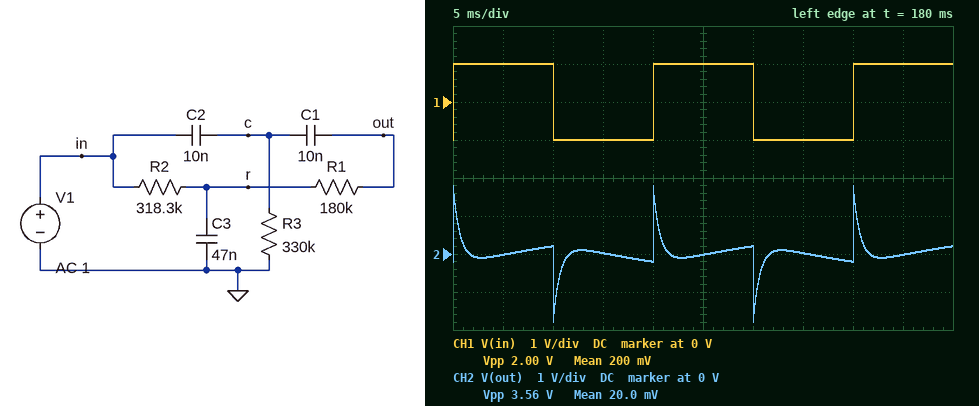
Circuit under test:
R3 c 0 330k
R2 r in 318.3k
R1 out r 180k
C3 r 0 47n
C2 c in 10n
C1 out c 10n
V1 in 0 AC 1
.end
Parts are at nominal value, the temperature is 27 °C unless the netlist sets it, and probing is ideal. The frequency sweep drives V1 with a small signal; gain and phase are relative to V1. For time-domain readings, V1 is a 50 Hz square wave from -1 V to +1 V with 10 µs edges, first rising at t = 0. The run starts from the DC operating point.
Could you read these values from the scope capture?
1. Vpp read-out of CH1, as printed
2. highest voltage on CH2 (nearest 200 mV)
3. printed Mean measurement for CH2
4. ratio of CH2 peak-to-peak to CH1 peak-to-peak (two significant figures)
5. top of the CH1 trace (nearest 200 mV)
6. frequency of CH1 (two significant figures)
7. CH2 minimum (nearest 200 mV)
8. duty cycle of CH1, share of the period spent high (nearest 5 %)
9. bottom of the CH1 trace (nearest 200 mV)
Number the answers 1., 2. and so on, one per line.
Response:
1. 2.00 V
2. 1.8 V
3. 20.0 mV
4. 1.8
5. 1.0 V
6. 50 Hz
7. -1.8 V
8. 50 %
9. -1.0 V
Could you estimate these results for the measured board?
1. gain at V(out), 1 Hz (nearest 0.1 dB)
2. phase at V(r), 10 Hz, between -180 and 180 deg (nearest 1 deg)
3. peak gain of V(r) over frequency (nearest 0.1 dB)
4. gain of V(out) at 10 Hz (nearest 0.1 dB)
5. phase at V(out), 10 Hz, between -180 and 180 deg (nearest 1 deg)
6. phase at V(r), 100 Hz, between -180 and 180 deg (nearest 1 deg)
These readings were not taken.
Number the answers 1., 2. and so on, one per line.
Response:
1. -0.1 dB
2. -46 deg
3. 0 dB
4. -4.5 dB
5. -52 deg
6. -49 deg
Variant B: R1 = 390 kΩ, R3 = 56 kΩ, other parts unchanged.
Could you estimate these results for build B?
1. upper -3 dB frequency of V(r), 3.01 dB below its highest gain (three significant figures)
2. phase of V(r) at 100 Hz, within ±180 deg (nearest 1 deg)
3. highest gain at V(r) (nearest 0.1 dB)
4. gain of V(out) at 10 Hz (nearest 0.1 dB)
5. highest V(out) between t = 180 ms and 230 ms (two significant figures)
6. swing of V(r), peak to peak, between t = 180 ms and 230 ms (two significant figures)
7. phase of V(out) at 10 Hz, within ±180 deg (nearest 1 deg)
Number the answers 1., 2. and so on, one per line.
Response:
1. 8.42 Hz
2. -68 deg
3. 0 dB
4. -4.2 dB
5. 1.9 V
6. 590 mV
7. -61 deg
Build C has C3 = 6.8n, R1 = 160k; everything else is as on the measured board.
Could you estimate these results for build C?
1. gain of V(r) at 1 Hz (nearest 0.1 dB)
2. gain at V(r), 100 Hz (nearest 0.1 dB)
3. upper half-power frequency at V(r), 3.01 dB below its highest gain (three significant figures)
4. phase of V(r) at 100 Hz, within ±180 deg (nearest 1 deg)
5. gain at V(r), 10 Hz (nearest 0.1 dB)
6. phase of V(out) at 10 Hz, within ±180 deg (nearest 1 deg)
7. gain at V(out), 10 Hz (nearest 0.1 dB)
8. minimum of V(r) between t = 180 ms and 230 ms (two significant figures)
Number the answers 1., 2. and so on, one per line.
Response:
1. 0 dB
2. -5.3 dB
3. 22.2 Hz
4. -20 deg
5. -1.1 dB
6. -21 deg
7. -1.5 dB
8. -720 mV
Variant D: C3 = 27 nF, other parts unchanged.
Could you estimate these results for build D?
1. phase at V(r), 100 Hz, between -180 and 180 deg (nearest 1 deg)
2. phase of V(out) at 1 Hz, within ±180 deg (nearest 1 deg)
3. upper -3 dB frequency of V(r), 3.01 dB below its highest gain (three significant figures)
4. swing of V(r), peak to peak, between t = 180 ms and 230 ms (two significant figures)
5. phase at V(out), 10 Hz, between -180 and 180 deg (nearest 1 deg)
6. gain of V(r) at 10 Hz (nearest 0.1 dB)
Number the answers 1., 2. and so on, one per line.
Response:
1. -44 deg
2. -5 deg
3. 11.8 Hz
4. 910 mV
5. -39 deg
6. -2.4 dB
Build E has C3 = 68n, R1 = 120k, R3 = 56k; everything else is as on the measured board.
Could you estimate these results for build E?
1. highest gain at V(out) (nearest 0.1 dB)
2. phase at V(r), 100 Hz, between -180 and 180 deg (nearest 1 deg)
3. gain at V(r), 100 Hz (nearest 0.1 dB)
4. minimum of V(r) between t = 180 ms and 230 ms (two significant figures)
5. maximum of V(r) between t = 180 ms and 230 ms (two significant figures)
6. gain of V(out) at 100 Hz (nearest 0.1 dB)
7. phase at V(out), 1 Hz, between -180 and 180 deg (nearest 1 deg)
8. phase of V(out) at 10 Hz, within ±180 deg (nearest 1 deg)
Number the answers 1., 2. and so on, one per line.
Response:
1. 0 dB
2. -57 deg
3. -24.3 dB
4. -200 mV
5. 200 mV
6. -18.3 dB
7. -9 deg
8. -61 deg
